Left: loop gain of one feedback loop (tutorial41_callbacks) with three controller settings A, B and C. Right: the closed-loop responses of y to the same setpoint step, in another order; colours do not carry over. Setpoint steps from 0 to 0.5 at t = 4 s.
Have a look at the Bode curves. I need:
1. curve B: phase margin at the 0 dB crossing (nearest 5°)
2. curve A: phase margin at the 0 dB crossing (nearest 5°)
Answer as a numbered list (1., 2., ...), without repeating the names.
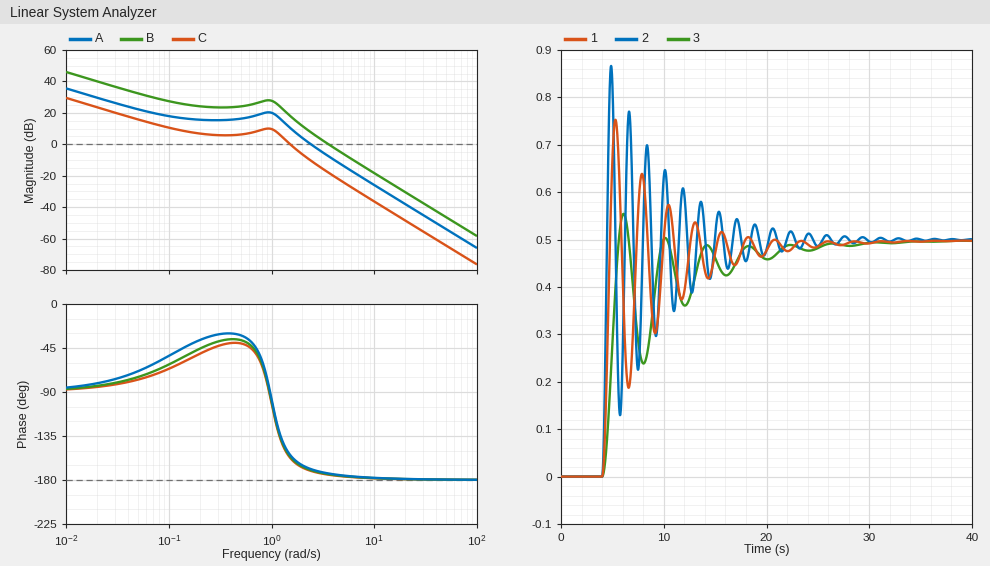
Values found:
1. 5°
2. 10°
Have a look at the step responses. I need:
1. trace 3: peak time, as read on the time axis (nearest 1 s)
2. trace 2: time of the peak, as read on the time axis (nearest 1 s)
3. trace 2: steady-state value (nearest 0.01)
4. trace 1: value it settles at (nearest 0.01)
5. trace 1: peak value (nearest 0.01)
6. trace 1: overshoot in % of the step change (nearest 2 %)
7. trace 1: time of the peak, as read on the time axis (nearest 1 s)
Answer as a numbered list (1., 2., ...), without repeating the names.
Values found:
1. 6 s
2. 5 s
3. 0.50
4. 0.50
5. 0.75
6. 50 %
7. 5 s
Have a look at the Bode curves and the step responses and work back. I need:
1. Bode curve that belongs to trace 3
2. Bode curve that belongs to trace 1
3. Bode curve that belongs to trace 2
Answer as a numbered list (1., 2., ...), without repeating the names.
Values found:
1. C
2. A
3. B
